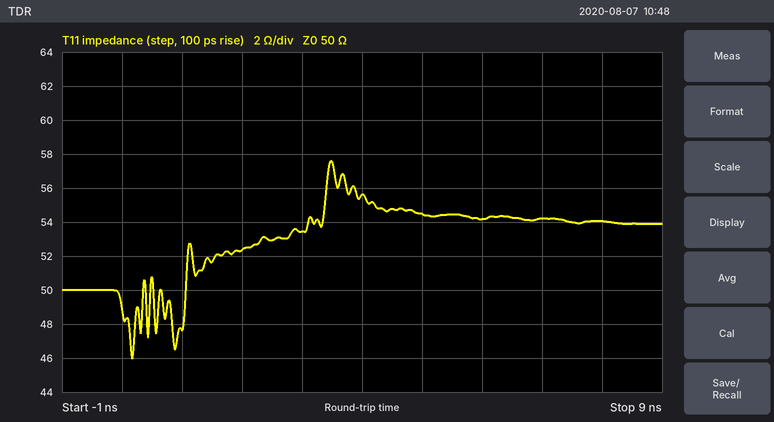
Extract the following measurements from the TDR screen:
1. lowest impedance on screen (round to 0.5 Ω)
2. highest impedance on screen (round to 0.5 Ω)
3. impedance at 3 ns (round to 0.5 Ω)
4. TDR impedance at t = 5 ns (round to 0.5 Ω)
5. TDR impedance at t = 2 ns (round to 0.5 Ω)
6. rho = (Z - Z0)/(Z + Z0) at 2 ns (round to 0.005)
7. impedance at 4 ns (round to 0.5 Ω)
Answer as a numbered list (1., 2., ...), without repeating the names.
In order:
1. 46.0 Ω
2. 57.5 Ω
3. 53.5 Ω
4. 54.5 Ω
5. 52.5 Ω
6. +0.025
7. 55.5 Ω
